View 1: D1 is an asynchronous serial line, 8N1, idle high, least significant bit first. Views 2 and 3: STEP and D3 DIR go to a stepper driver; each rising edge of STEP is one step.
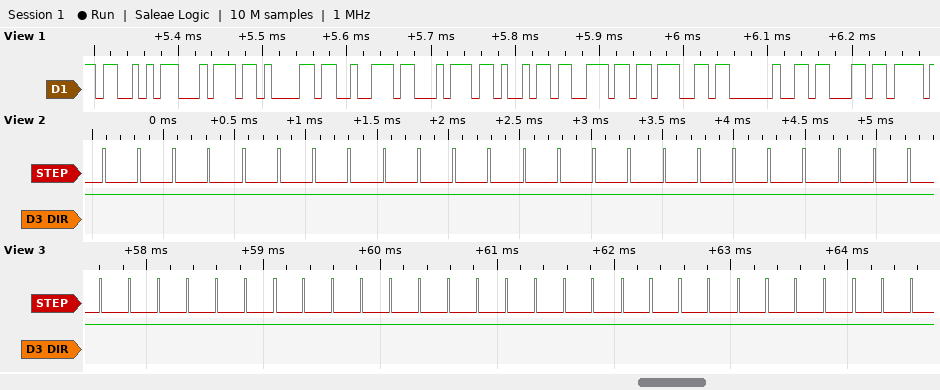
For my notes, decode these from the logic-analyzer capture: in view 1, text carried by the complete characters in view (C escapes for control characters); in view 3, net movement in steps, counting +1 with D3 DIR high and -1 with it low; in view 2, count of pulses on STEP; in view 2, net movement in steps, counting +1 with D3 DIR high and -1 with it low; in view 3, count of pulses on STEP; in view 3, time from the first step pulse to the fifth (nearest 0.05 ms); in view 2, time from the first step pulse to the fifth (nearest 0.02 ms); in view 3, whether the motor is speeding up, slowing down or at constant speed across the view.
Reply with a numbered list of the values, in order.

1. "Starting c"
2. +29
3. 24
4. +24
5. 29
6. 1.00 ms
7. 0.98 ms
8. constant speed
